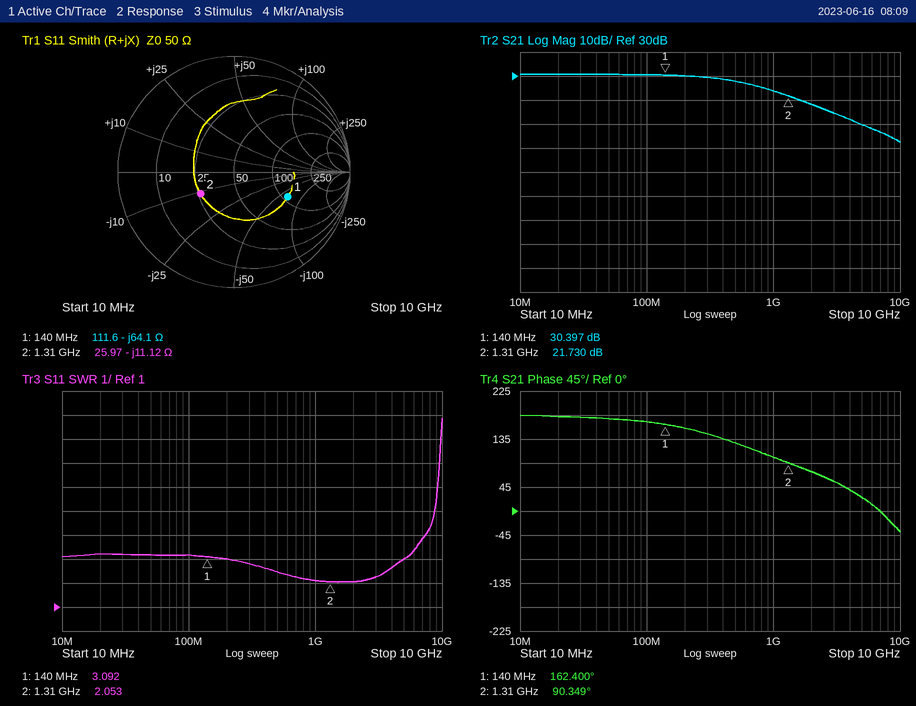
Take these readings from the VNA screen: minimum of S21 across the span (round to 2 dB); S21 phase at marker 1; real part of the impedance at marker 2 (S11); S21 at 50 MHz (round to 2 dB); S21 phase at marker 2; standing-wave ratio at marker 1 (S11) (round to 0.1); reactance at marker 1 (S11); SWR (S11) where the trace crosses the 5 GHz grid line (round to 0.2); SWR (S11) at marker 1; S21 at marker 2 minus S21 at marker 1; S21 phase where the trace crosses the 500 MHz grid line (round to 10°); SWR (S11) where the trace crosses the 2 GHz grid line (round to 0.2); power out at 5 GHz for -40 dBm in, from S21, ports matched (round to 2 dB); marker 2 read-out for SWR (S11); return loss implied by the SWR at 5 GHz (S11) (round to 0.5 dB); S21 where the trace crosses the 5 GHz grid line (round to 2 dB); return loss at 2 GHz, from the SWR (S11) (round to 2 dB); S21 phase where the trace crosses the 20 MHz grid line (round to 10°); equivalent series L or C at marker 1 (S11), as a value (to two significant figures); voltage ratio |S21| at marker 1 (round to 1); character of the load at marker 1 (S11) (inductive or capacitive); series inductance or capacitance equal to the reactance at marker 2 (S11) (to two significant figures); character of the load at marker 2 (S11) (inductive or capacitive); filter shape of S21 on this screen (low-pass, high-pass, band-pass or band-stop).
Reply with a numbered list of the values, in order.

1. 2 dB
2. 162.400°
3. 25.97 Ω
4. 30 dB
5. 90.349°
6. 3.1
7. -64.1 Ω
8. 3.0
9. 3.092
10. -8.667 dB
11. 130°
12. 2.0
13. -30 dBm
14. 2.053
15. 6.0 dB
16. 10 dB
17. 10 dB
18. 180°
19. 18 pF
20. 33
21. capacitive
22. 11 pF
23. capacitive
24. low-pass
